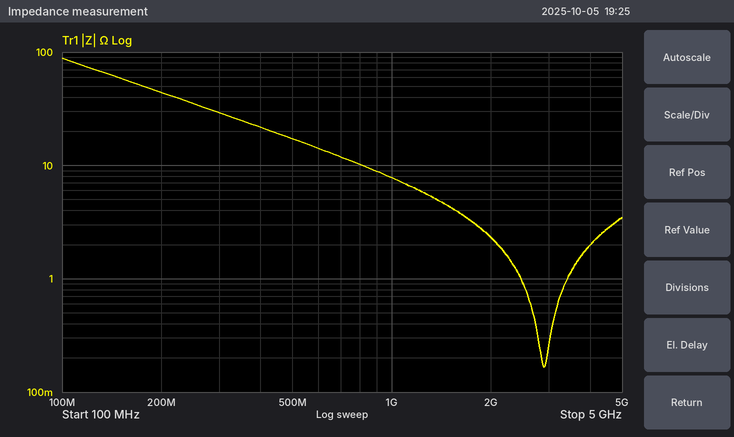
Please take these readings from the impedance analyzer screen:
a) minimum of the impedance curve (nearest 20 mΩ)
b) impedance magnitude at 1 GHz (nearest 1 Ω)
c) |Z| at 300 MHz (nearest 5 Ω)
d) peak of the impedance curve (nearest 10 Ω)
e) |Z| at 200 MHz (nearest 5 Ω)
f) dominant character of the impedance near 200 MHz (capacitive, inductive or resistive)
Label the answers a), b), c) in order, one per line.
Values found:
a) 160 mΩ
b) 8 Ω
c) 30 Ω
d) 90 Ω
e) 45 Ω
f) capacitive
